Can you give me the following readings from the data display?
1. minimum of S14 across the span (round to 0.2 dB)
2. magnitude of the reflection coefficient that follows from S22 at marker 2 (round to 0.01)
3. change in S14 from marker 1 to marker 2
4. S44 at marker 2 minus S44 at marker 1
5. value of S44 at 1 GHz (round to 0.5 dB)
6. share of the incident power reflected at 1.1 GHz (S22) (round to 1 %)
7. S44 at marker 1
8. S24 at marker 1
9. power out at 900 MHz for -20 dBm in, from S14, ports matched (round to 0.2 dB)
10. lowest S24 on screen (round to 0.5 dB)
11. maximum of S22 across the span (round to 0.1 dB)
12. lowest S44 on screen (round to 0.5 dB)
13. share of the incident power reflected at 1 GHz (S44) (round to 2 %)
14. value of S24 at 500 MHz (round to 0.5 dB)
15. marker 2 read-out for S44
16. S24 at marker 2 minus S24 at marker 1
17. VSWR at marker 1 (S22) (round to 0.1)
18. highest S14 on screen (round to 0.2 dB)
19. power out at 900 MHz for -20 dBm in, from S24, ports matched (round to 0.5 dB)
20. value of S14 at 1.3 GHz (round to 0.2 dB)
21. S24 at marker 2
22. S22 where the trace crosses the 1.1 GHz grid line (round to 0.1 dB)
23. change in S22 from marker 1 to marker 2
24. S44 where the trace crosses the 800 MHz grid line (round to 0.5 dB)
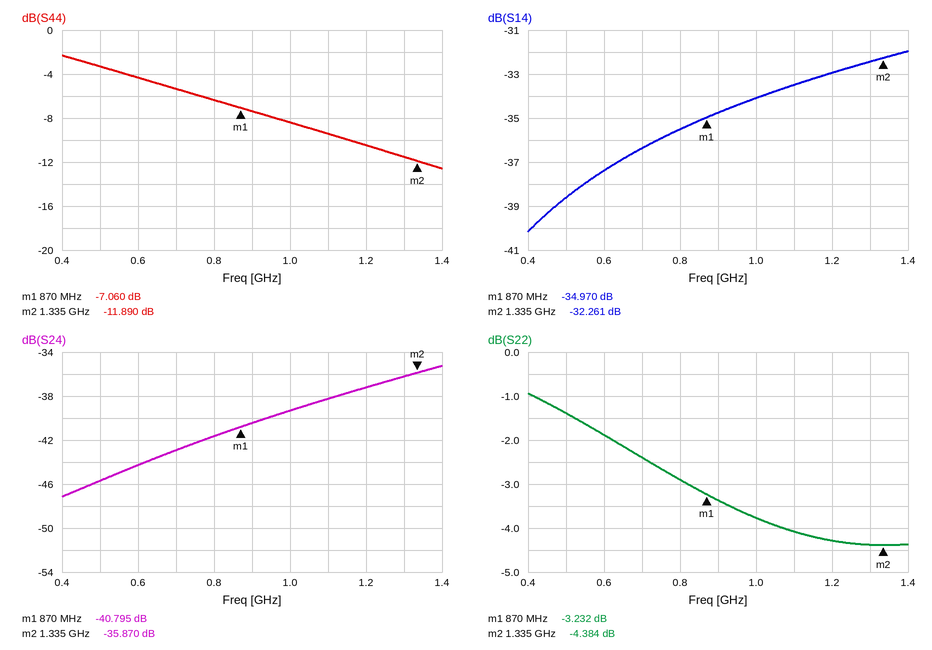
-40.2 dB
0.60
2.709 dB
-4.830 dB
-8.5 dB
39 %
-7.060 dB
-40.795 dB
-54.8 dBm
-47.0 dB
-0.9 dB
-12.5 dB
14 %
-45.5 dB
-11.890 dB
4.925 dB
5.4
-32.0 dB
-60.5 dBm
-32.4 dB
-35.870 dB
-4.1 dB
-1.152 dB
-6.5 dB
